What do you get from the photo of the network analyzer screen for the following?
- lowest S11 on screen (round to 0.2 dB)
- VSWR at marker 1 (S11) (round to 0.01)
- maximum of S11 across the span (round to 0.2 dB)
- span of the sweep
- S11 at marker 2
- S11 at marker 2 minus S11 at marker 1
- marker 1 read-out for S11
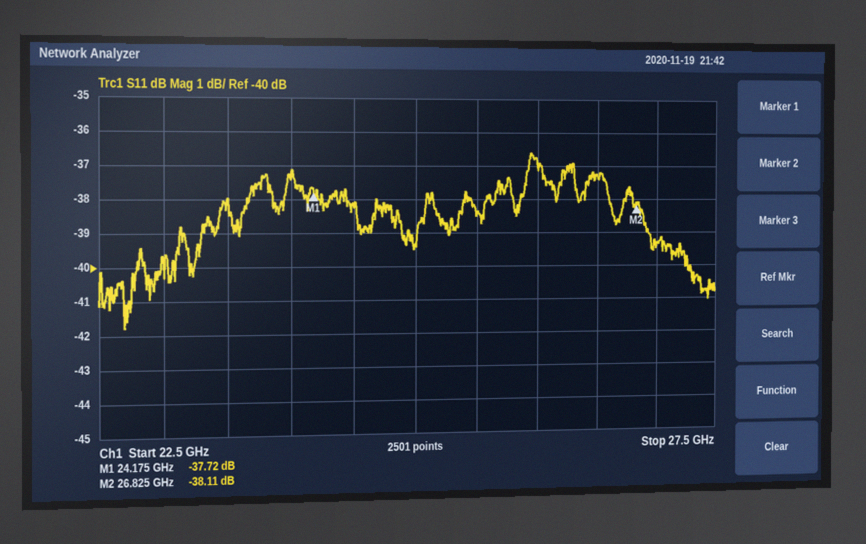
-41.8 dB
1.03
-36.6 dB
5 GHz
-38.11 dB
-0.39 dB
-37.72 dB
